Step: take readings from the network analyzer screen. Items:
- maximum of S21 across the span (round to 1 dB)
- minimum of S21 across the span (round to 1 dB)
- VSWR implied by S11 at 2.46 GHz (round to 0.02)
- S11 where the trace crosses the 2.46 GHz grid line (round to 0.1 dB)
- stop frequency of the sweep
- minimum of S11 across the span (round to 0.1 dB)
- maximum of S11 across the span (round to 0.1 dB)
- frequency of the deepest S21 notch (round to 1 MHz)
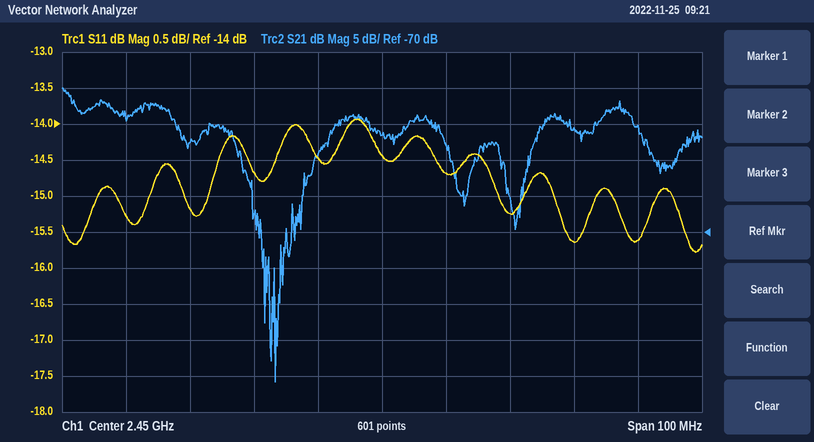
-50 dB
-91 dB
1.46
-14.7 dB
2.5 GHz
-15.8 dB
-13.9 dB
2.433 GHz
